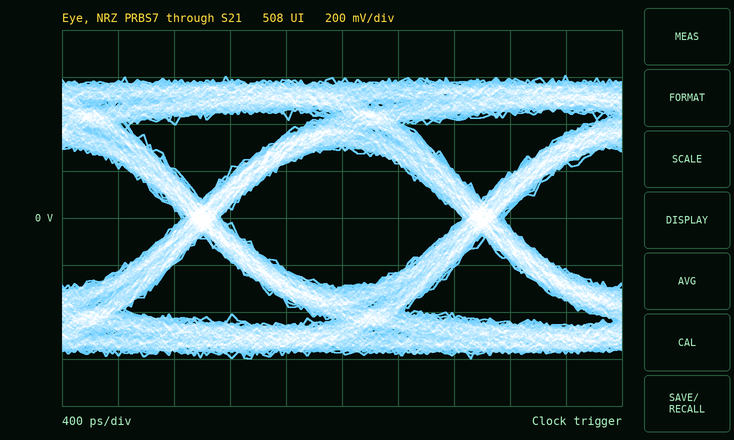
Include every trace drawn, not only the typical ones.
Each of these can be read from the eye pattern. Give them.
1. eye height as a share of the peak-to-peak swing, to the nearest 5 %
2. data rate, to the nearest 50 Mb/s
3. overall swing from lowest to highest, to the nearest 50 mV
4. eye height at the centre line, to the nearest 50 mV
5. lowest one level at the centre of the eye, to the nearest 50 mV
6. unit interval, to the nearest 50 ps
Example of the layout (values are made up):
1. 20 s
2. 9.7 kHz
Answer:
1. 50 %
2. 500 Mb/s
3. 1.20 V
4. 600 mV
5. 300 mV
6. 2.00 ns
